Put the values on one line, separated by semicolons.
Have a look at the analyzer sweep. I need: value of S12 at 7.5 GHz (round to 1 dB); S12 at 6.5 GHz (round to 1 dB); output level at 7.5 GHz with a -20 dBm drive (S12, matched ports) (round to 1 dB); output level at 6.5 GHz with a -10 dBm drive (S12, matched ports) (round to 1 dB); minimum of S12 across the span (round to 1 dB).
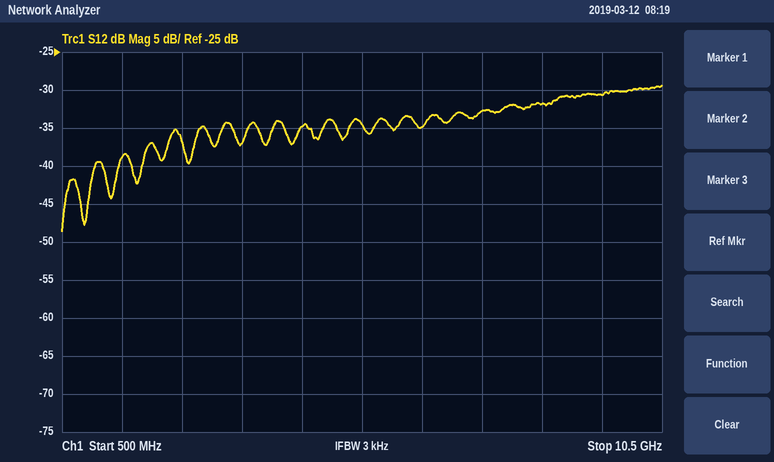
-33 dB; -35 dB; -53 dBm; -45 dBm; -49 dB
